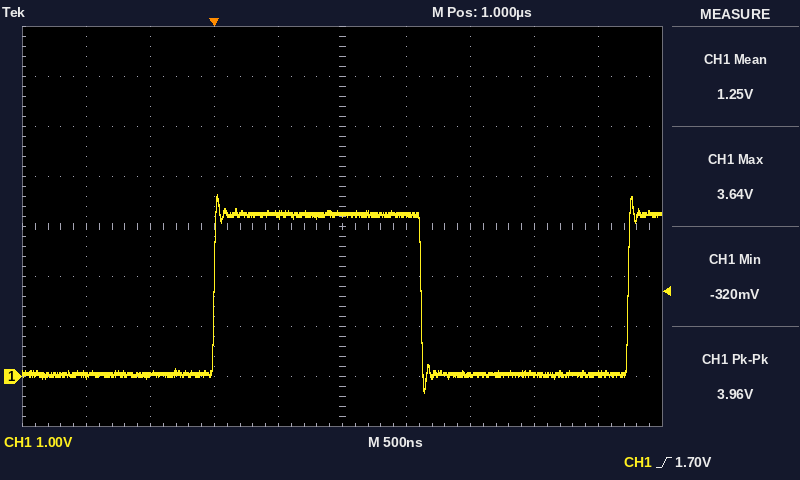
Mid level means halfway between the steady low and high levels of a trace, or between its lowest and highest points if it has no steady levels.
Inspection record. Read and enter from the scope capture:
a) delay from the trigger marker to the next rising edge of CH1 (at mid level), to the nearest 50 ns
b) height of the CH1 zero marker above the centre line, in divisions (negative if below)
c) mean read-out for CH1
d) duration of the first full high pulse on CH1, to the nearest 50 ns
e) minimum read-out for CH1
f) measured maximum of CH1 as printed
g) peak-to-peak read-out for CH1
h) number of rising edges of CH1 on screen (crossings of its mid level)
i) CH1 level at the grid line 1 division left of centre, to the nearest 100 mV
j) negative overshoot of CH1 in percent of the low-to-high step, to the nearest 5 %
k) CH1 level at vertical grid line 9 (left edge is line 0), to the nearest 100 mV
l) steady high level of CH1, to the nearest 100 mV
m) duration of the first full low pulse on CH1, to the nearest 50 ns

3.25 µs
-3.0 div
1.25 V
1.60 µs
-320 mV
3.64 V
3.96 V
2
3.2 V
10 %
100 mV
3.2 V
1.60 µs
